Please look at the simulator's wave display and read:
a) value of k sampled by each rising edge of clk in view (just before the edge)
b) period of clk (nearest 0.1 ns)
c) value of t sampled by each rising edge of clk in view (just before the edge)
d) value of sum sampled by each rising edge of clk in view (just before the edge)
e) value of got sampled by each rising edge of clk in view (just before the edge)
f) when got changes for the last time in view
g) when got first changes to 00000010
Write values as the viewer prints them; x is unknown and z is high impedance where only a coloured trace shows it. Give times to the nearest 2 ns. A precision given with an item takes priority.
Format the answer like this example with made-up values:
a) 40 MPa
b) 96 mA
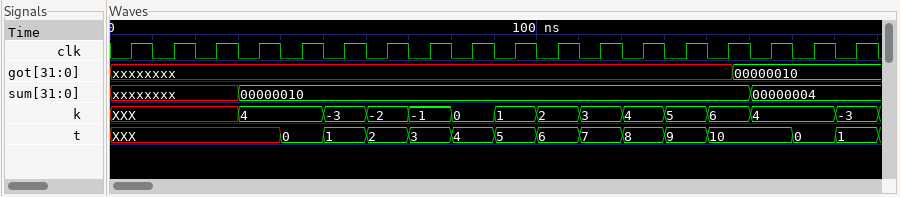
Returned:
a) XXX, XXX, XXX, 4, 4, -3, -2, -1, 0, 1, 2, 3, 4, 5, 6, 4, 4, -3
b) 10 ns
c) XXX, XXX, XXX, XXX, 0, 1, 2, 3, 4, 5, 6, 7, 8, 9, 10, 10, 0, 1
d) xxxxxxxx, xxxxxxxx, xxxxxxxx, 00000010, 00000010, 00000010, 00000010, 00000010, 00000010, 00000010, 00000010, 00000010, 00000010, 00000010, 00000010, 00000004, 00000004, 00000004
e) xxxxxxxx, xxxxxxxx, xxxxxxxx, xxxxxxxx, xxxxxxxx, xxxxxxxx, xxxxxxxx, xxxxxxxx, xxxxxxxx, xxxxxxxx, xxxxxxxx, xxxxxxxx, xxxxxxxx, xxxxxxxx, xxxxxxxx, 00000010, 00000010, 00000010
f) 146 ns
g) 146 ns
